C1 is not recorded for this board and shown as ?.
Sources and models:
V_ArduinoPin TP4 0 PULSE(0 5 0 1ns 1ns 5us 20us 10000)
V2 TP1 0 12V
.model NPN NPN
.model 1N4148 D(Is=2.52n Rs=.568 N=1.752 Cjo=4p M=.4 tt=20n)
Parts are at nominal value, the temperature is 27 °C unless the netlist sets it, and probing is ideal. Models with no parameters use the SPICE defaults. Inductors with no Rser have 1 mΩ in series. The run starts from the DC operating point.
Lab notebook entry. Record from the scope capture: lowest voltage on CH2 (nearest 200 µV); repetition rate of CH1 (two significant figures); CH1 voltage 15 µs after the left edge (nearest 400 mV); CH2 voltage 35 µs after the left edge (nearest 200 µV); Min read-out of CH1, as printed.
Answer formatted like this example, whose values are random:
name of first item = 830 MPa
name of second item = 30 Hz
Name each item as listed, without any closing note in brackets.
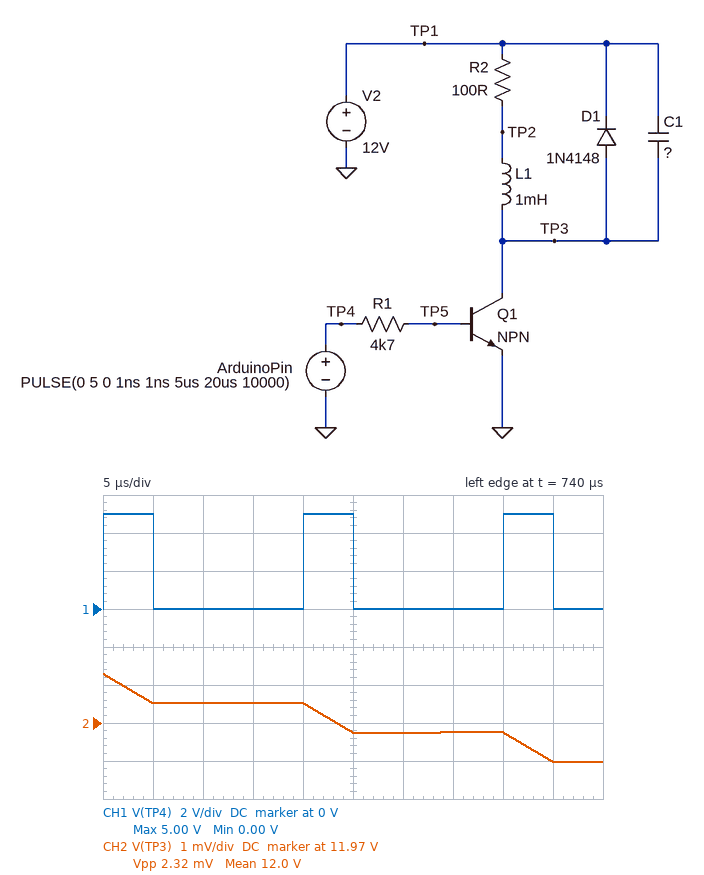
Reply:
lowest voltage on CH2 = 11.9690 V
repetition rate of CH1 = 50 kHz
CH1 voltage 15 µs after the left edge = 0 V
CH2 voltage 35 µs after the left edge = 11.9698 V
Min read-out of CH1, as printed = 0.00 V
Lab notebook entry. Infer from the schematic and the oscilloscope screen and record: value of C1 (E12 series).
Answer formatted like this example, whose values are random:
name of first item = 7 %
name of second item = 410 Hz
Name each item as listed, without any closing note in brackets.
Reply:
value of C1 = 560 µF
